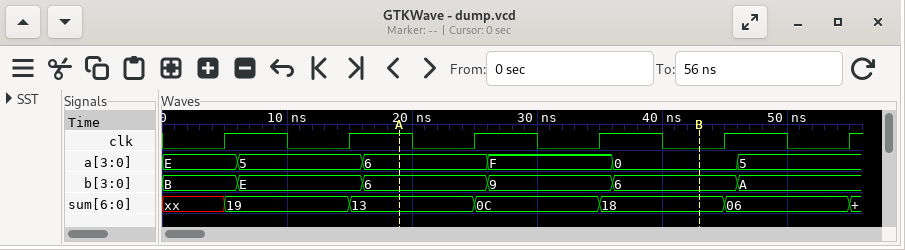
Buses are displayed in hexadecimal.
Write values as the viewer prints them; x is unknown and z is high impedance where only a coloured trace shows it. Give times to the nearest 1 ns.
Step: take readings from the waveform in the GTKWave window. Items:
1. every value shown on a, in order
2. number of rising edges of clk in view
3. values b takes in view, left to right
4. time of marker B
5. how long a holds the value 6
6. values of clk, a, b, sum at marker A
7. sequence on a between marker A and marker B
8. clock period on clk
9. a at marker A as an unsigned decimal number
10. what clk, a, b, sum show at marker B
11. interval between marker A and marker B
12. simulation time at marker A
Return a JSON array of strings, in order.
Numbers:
["E, 5, 6, F, 0, 5", "6", "B, E, 6, 9, 6, A", "43 ns", "10 ns", "clk=1, a=6, b=6, sum=13", "6, F, 0", "10 ns", "6", "clk=0, a=0, b=6, sum=18", "24 ns", "19 ns"]
